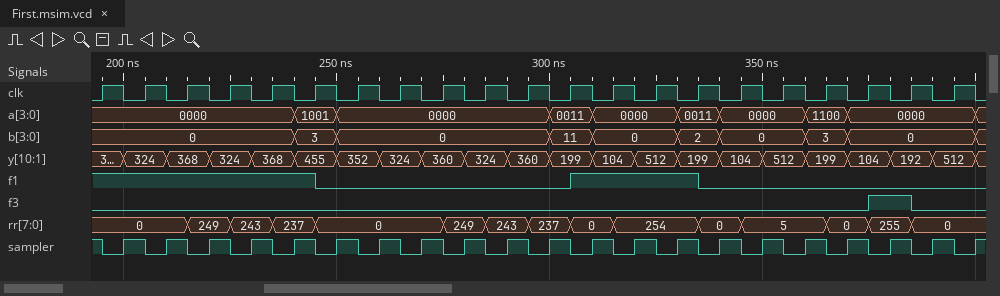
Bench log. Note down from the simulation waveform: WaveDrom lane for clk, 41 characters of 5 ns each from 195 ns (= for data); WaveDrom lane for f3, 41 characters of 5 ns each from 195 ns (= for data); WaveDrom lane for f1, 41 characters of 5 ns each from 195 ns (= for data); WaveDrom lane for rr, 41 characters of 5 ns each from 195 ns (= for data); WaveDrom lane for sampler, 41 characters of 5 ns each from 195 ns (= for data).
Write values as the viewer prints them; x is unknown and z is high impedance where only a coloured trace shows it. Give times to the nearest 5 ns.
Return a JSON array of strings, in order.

["{name: 'clk', wave: '10101010101010101010101010101010101010101'}", "{name: 'f3', wave: '0...................................1.0..'}", "{name: 'f1', wave: '1.........0...........1.....0............'}", "{name: 'rr', wave: '=...=.=.=.=.....=.=.=.=.=...=.=...=.=.=..', data: '0 249 243 237 0 249 243 237 0 254 0 5 0 255 0'}", "{name: 'sampler', wave: '01010101010101010101010101010101010101010'}"]
